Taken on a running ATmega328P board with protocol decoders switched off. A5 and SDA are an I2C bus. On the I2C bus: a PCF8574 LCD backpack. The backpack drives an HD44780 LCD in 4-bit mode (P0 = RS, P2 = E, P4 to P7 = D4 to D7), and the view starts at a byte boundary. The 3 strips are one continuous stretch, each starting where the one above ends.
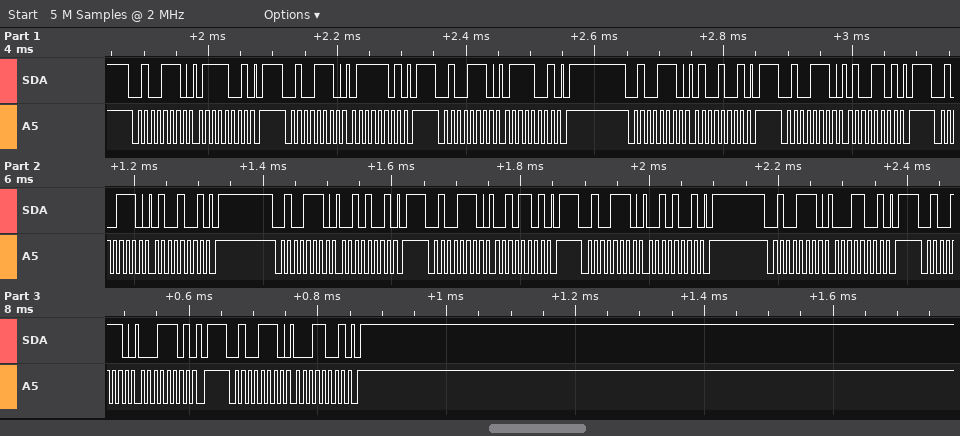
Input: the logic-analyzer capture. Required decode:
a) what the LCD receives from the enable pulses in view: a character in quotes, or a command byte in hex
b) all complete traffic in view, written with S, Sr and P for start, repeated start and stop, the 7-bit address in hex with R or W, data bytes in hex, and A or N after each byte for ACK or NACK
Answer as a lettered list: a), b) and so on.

a) 't' '!'
b) S 27W A 79 A P S 27W A 7D A P S 27W A 79 A P S 27W A 49 A P S 27W A 4D A P S 27W A 49 A P S 27W A 29 A P S 27W A 2D A P S 27W A 29 A P S 27W A 19 A P S 27W A 1D A P S 27W A 19 A P
